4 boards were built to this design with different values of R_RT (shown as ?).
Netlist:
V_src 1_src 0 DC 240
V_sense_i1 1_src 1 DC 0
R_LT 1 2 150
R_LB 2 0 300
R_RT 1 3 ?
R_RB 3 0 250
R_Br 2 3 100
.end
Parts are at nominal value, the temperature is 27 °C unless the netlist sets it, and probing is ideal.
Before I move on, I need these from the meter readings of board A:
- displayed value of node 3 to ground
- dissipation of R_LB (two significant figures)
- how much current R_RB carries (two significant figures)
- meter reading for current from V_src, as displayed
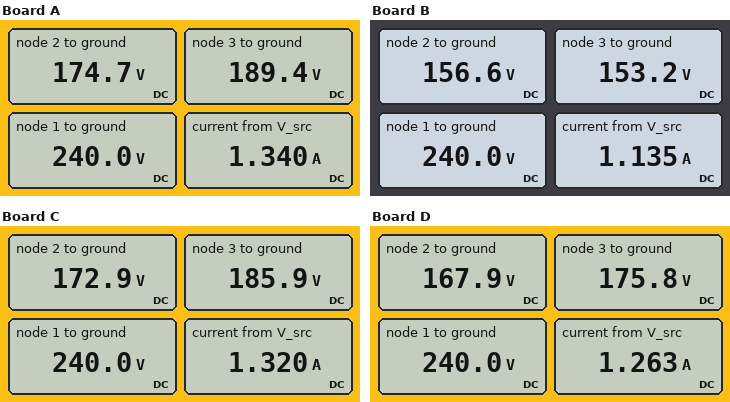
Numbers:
189.4 V
100 W
760 mA
1.340 A
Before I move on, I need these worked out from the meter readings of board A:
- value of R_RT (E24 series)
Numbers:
56 Ω
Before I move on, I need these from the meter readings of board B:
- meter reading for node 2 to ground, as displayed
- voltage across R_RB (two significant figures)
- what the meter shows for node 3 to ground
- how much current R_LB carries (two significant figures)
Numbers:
156.6 V
150 V
153.2 V
520 mA
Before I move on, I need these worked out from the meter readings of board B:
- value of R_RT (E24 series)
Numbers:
150 Ω
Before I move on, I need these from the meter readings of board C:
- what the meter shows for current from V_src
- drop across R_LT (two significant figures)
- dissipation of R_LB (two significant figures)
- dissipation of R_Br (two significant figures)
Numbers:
1.320 A
67 V
100 W
1.7 W
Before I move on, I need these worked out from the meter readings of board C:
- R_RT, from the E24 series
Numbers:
62 Ω
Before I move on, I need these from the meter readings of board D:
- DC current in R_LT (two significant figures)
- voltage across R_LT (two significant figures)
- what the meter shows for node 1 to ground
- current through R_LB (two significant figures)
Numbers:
480 mA
72 V
240.0 V
560 mA
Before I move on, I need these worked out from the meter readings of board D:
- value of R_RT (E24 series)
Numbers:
82 Ω
